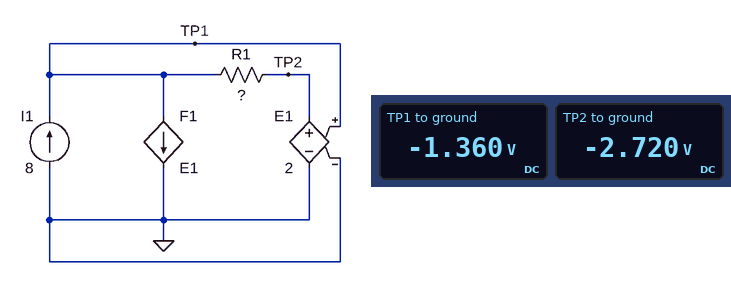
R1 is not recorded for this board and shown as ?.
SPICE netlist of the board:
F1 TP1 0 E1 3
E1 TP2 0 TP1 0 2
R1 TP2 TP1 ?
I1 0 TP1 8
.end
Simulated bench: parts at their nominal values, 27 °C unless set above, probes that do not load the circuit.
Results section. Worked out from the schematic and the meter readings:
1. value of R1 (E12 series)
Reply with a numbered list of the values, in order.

1. 0.68 Ω
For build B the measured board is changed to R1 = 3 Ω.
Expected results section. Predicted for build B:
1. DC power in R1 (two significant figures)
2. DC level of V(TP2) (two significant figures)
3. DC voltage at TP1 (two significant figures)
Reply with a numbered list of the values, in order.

1. 12 W
2. -12 V
3. -6.0 V
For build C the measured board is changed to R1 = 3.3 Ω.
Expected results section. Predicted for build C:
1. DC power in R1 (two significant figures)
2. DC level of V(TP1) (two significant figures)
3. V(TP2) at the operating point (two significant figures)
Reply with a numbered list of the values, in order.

1. 13 W
2. -6.6 V
3. -13 V
